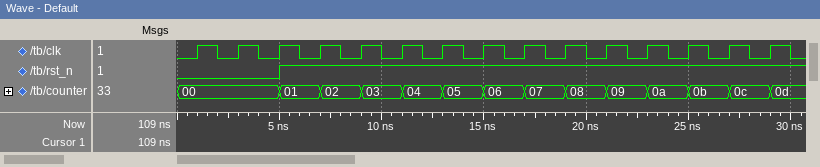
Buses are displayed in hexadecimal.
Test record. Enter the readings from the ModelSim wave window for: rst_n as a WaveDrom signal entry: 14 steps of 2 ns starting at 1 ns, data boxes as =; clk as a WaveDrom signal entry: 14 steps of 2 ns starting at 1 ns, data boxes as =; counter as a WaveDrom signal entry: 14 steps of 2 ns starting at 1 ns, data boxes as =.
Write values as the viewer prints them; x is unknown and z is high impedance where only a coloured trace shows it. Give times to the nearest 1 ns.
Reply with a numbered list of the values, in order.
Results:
1. {name: 'rst_n', wave: '0.1...........'}
2. {name: 'clk', wave: 'p.............'}
3. {name: 'counter', wave: '=.============', data: '00 01 02 03 04 05 06 07 08 09 0a 0b 0c'}
